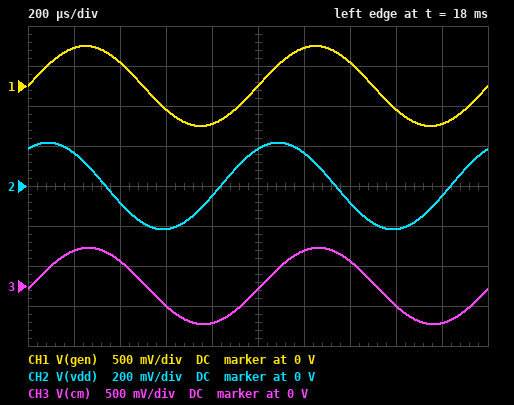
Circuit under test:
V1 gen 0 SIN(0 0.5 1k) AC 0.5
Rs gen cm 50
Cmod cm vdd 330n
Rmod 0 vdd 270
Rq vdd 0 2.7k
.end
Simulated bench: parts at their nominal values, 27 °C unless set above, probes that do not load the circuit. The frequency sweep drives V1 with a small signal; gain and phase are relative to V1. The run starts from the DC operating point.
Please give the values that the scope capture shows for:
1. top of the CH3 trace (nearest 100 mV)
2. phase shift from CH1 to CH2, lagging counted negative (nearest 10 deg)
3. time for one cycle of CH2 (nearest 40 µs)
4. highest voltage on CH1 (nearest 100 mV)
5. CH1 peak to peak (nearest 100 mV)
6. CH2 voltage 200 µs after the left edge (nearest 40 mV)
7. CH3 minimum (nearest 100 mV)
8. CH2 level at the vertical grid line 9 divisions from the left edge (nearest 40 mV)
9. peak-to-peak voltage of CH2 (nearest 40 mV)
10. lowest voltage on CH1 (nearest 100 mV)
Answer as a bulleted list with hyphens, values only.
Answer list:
- 500 mV
- 60 deg
- 1.00 ms
- 500 mV
- 1.0 V
- 160 mV
- -500 mV
- -40 mV
- 440 mV
- -500 mV
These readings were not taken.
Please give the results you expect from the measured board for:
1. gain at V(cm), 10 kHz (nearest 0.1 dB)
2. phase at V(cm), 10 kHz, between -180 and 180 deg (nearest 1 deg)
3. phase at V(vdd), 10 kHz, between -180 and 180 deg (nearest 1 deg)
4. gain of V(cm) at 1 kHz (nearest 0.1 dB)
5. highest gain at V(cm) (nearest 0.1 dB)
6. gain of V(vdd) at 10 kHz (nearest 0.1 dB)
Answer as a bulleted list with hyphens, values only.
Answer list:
- -1.6 dB
- -2 deg
- 9 deg
- -0.4 dB
- 0 dB
- -1.7 dB
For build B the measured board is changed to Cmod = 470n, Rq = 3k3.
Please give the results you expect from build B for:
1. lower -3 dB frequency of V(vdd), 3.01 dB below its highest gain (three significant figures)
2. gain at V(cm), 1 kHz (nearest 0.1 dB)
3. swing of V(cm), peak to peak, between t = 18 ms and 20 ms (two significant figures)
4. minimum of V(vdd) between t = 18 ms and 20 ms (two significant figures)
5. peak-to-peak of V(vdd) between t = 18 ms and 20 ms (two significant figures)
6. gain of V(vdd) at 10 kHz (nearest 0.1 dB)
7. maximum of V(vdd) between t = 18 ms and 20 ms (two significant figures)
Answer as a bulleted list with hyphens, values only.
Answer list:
- 1.13 kHz
- -0.6 dB
- 930 mV
- -280 mV
- 550 mV
- -1.6 dB
- 280 mV
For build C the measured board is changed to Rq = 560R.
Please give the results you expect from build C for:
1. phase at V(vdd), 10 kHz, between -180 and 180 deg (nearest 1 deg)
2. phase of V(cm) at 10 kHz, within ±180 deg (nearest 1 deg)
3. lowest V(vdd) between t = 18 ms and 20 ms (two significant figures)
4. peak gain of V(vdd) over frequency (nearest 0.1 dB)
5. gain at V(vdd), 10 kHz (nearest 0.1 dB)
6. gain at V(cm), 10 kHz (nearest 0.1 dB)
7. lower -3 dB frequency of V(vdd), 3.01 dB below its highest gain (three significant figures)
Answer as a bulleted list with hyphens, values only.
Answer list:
- 12 deg
- -3 deg
- -170 mV
- -2.1 dB
- -2.3 dB
- -2.0 dB
- 2.08 kHz
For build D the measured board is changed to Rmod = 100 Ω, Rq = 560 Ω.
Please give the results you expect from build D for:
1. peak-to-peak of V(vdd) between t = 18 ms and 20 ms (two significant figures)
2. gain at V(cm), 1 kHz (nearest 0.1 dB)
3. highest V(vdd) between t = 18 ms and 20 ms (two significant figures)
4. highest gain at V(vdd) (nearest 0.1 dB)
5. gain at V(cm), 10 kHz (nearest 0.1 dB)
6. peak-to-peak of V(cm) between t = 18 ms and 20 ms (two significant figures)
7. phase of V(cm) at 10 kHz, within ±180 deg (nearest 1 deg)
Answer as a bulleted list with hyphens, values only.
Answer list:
- 170 mV
- -0.2 dB
- 85 mV
- -4.0 dB
- -3.3 dB
- 980 mV
- -10 deg
